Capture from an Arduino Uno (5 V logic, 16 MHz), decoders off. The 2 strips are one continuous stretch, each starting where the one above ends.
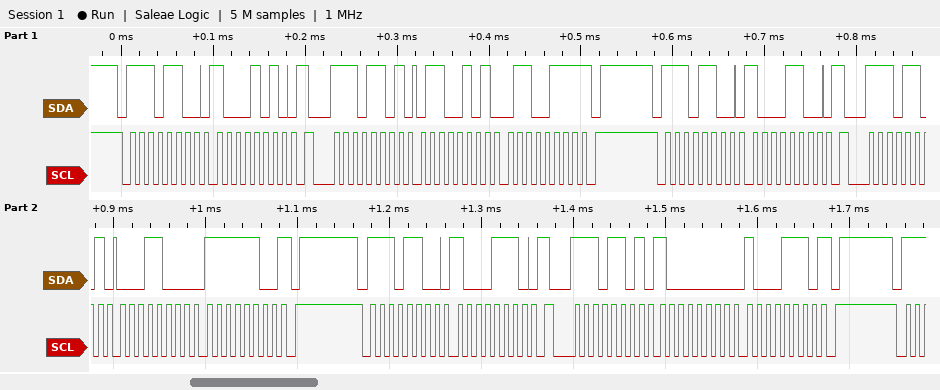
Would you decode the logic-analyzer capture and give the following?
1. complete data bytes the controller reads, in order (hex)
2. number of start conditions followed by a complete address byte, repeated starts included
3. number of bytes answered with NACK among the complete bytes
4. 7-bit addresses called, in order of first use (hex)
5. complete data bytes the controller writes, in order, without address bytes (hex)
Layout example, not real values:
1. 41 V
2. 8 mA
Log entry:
1. 65 67 18 FC 80 8E
2. 6
3. 3
4. 0x76
5. 8A 8C 8E
